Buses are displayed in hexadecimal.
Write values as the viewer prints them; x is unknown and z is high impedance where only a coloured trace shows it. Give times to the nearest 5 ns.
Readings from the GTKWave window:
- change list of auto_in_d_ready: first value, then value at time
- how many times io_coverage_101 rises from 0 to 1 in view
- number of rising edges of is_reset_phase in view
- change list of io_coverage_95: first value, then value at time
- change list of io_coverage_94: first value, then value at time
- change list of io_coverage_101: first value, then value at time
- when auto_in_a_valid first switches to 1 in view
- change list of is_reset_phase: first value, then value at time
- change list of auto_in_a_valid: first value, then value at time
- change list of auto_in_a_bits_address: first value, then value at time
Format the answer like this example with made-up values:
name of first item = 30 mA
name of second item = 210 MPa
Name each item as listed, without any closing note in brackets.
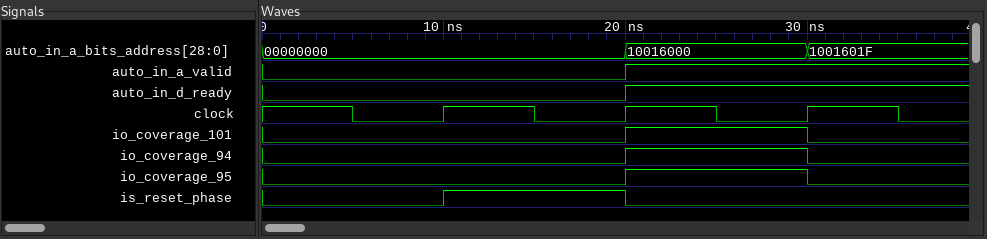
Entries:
change list of auto_in_d_ready: first value, then value at time = 0, 1 at 20 ns
how many times io_coverage_101 rises from 0 to 1 in view = 1
number of rising edges of is_reset_phase in view = 1
change list of io_coverage_95: first value, then value at time = 0, 1 at 20 ns, 0 at 30 ns
change list of io_coverage_94: first value, then value at time = 0, 1 at 20 ns, 0 at 30 ns
change list of io_coverage_101: first value, then value at time = 0, 1 at 20 ns, 0 at 30 ns
when auto_in_a_valid first switches to 1 in view = 20 ns
change list of is_reset_phase: first value, then value at time = 0, 1 at 10 ns, 0 at 20 ns
change list of auto_in_a_valid: first value, then value at time = 0, 1 at 20 ns
change list of auto_in_a_bits_address: first value, then value at time = 00000000, 10016000 at 20 ns, 1001601F at 30 ns
